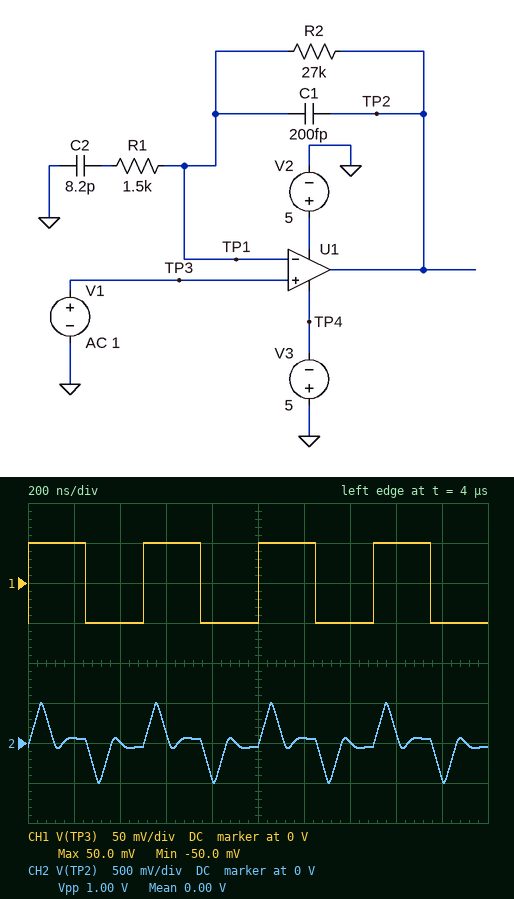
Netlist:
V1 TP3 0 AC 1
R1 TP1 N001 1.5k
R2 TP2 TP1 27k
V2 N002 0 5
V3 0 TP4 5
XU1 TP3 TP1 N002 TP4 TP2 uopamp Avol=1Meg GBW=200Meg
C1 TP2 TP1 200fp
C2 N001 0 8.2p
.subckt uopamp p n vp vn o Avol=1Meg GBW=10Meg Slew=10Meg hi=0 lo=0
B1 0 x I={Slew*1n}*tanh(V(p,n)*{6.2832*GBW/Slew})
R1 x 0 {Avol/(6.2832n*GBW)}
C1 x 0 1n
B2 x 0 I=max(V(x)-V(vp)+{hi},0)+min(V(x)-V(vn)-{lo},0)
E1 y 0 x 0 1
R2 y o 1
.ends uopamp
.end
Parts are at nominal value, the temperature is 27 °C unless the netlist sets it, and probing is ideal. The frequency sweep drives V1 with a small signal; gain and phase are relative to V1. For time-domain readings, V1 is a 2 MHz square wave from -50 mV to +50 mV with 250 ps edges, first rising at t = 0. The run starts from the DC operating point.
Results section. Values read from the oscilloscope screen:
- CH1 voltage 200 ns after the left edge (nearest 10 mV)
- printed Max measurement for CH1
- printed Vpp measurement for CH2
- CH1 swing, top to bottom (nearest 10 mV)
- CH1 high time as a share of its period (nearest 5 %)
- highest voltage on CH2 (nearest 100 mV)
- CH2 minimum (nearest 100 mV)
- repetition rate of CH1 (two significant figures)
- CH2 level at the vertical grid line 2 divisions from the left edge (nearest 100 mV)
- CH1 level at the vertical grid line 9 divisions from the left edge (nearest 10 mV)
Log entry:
50 mV
50.0 mV
1.00 V
100 mV
50 %
500 mV
-500 mV
2.0 MHz
0 V
-50 mV
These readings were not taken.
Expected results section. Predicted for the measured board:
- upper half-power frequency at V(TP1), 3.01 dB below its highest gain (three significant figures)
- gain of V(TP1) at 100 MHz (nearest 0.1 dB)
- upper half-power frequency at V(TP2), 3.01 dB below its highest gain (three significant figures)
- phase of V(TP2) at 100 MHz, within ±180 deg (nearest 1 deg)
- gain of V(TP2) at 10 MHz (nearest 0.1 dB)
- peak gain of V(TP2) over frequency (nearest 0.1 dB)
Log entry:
14.0 MHz
-11.2 dB
17.3 MHz
-81 deg
22.3 dB
22.3 dB
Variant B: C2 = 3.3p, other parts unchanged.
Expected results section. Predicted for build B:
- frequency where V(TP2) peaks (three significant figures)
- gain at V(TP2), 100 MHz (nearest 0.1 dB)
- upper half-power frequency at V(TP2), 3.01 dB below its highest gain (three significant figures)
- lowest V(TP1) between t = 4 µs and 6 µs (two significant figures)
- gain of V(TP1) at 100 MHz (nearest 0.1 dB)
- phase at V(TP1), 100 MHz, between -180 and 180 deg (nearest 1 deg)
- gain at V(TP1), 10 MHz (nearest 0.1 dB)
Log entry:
15.6 MHz
3.8 dB
26.1 MHz
-69 mV
-11.0 dB
-32 deg
1.7 dB
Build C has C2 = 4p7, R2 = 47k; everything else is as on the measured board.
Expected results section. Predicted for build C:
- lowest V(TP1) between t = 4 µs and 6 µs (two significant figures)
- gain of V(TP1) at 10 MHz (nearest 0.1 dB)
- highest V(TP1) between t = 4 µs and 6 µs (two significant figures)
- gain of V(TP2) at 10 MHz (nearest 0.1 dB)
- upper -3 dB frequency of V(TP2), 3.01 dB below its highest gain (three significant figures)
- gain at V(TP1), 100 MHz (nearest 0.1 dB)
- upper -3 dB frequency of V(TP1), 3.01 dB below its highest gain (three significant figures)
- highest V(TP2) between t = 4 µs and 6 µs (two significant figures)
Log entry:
-72 mV
1.5 dB
72 mV
22.9 dB
16.8 MHz
-11.3 dB
13.6 MHz
510 mV
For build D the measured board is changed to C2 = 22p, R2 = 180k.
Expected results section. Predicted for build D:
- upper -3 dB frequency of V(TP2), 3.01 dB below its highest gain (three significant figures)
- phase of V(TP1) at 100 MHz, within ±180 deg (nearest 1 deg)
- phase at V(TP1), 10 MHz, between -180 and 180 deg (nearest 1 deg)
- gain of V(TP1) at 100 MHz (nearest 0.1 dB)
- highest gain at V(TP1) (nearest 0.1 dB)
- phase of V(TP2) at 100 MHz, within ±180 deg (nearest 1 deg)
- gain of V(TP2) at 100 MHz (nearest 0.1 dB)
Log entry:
3.98 MHz
-12 deg
-35 deg
-11.4 dB
2.2 dB
-86 deg
3.4 dB
